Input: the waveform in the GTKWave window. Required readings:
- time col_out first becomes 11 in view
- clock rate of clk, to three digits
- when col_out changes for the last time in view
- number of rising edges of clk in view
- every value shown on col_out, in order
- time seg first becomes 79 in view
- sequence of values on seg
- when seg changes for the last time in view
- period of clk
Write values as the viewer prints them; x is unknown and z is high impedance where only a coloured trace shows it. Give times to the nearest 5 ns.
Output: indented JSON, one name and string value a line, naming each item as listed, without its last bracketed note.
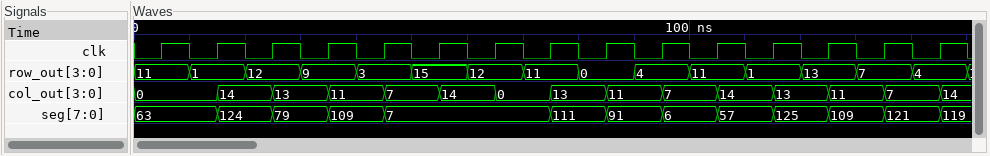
{
  "time col_out first becomes 11 in view": "35 ns",
  "clock rate of clk, to three digits": "100 MHz",
  "when col_out changes for the last time in view": "145 ns",
  "number of rising edges of clk in view": "15",
  "every value shown on col_out, in order": "0, 14, 13, 11, 7, 14, 0, 13, 11, 7, 14, 13, 11, 7, 14",
  "time seg first becomes 79 in view": "25 ns",
  "sequence of values on seg": "63, 124, 79, 109, 7, 111, 91, 6, 57, 125, 109, 121, 119",
  "when seg changes for the last time in view": "145 ns",
  "period of clk": "10 ns"
}
